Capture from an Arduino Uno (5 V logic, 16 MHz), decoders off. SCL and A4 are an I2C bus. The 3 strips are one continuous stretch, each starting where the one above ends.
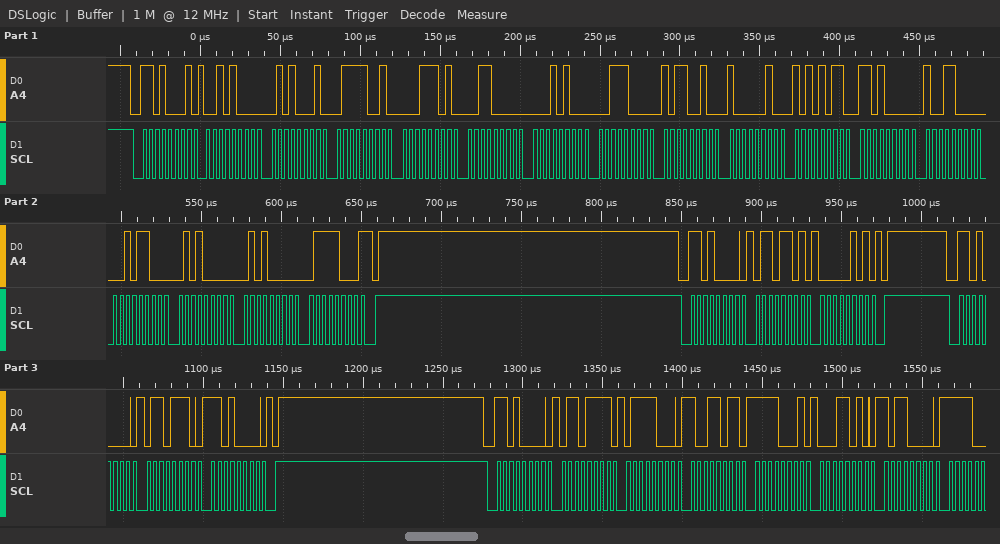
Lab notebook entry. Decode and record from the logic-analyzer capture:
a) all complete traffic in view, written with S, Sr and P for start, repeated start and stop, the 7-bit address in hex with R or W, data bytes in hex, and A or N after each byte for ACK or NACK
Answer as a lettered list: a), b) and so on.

a) S 68R A 28 A 51 A 79 A 1D A 30 A 14 A 38 A B2 A 82 A AB A D0 A 98 A 2C A 50 A 50 A 78 N P S 68W A 6D A 05 A P S 68W A 6E A D0 A P S 68W A 6F A 78 A 9B A F1 A 1A A B0 A
